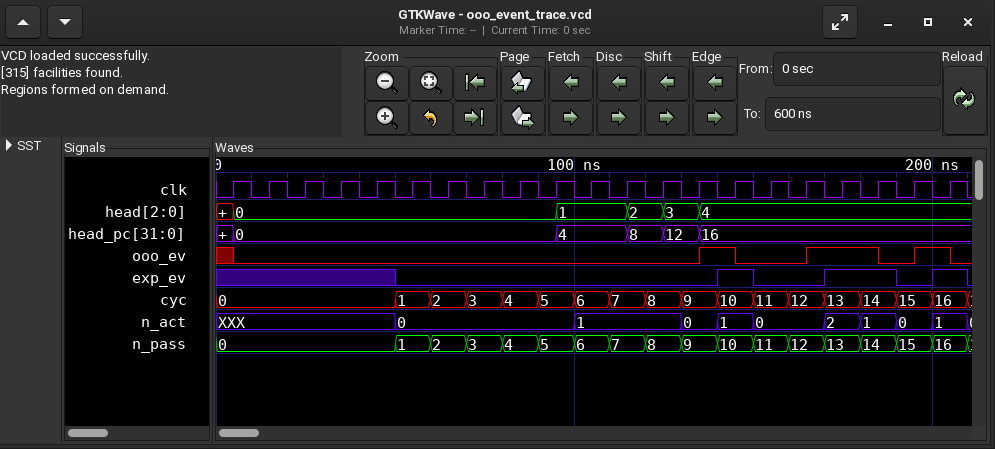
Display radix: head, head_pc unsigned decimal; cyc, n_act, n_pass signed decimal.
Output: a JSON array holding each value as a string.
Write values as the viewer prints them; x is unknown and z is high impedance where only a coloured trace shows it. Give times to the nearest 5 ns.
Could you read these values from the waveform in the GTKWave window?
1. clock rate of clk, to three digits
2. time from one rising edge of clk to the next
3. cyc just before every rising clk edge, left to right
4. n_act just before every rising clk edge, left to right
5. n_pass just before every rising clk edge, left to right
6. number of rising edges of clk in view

["100 MHz", "10 ns", "0, 0, 0, 0, 0, 1, 2, 3, 4, 5, 6, 7, 8, 9, 10, 11, 12, 13, 14, 15, 16", "XXX, XXX, XXX, XXX, XXX, 0, 0, 0, 0, 0, 1, 1, 1, 0, 1, 0, 0, 2, 1, 0, 1", "0, 0, 0, 0, 0, 1, 2, 3, 4, 5, 6, 7, 8, 9, 10, 11, 12, 13, 14, 15, 16", "21"]
